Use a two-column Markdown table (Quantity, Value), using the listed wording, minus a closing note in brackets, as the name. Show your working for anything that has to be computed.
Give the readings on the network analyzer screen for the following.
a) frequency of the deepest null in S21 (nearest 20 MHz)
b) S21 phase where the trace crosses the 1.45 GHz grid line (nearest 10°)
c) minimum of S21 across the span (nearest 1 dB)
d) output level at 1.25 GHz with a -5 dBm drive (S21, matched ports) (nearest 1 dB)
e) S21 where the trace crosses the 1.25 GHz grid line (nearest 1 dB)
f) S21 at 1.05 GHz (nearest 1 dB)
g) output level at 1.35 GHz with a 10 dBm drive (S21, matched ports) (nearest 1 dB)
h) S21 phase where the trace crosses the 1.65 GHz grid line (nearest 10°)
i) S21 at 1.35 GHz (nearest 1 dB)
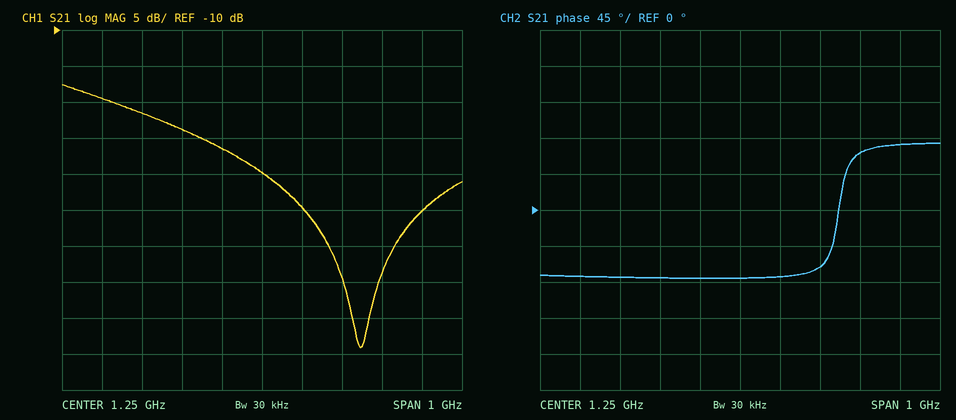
| Quantity | Value |
|---|---|
| frequency of the deepest null in S21 | 1.50 GHz |
| S21 phase where the trace crosses the 1.45 GHz grid line | -70° |
| minimum of S21 across the span | -54 dB |
| output level at 1.25 GHz with a -5 dBm drive (S21, matched ports) | -5 dBm + (-30 dB) = -35 dBm |
| S21 where the trace crosses the 1.25 GHz grid line | -30 dB |
| S21 at 1.05 GHz | -24 dB |
| output level at 1.35 GHz with a 10 dBm drive (S21, matched ports) | 10 dBm + (-35 dB) = -25 dBm |
| S21 phase where the trace crosses the 1.65 GHz grid line | 80° |
| S21 at 1.35 GHz | -35 dB |
